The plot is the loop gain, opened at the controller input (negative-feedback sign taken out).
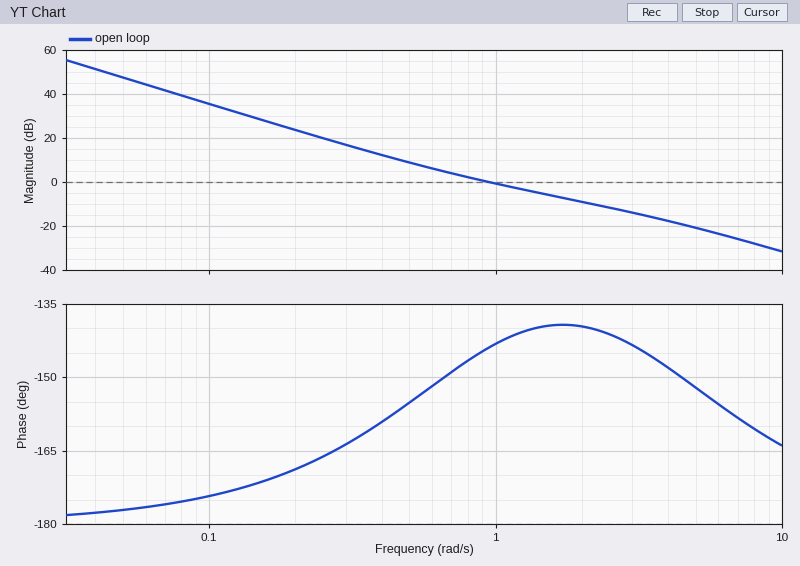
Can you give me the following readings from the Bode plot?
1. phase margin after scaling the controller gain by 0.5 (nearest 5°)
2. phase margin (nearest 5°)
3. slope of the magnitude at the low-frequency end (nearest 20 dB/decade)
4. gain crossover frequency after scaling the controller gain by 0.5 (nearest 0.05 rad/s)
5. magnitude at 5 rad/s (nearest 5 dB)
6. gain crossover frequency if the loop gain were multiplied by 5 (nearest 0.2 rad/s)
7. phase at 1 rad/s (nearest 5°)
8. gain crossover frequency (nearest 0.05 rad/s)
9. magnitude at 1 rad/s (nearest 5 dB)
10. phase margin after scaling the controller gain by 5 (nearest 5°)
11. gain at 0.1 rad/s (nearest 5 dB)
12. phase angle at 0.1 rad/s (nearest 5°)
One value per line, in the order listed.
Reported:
30°
35°
-40 dB/decade
0.60 rad/s
-20 dB
3.0 rad/s
-145°
0.95 rad/s
0 dB
35°
35 dB
-175°
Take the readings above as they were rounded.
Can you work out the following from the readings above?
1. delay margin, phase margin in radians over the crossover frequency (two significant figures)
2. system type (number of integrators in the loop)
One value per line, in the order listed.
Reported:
0.64 s
2
